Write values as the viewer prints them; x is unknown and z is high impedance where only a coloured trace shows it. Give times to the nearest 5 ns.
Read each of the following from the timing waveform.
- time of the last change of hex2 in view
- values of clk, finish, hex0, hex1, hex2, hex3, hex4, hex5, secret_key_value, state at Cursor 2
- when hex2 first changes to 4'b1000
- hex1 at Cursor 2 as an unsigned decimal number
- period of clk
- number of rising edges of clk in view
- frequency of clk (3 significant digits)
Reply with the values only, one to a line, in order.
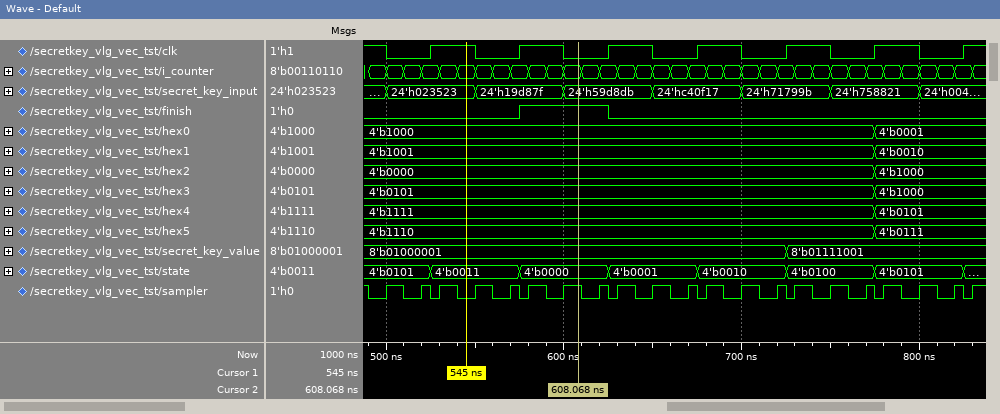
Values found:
775 ns
clk=0, finish=1, hex0=4'b1000, hex1=4'b1001, hex2=4'b0000, hex3=4'b0101, hex4=4'b1111, hex5=4'b1110, secret_key_value=8'b01000001, state=4'b0000
775 ns
9
50 ns
7
20.0 MHz
